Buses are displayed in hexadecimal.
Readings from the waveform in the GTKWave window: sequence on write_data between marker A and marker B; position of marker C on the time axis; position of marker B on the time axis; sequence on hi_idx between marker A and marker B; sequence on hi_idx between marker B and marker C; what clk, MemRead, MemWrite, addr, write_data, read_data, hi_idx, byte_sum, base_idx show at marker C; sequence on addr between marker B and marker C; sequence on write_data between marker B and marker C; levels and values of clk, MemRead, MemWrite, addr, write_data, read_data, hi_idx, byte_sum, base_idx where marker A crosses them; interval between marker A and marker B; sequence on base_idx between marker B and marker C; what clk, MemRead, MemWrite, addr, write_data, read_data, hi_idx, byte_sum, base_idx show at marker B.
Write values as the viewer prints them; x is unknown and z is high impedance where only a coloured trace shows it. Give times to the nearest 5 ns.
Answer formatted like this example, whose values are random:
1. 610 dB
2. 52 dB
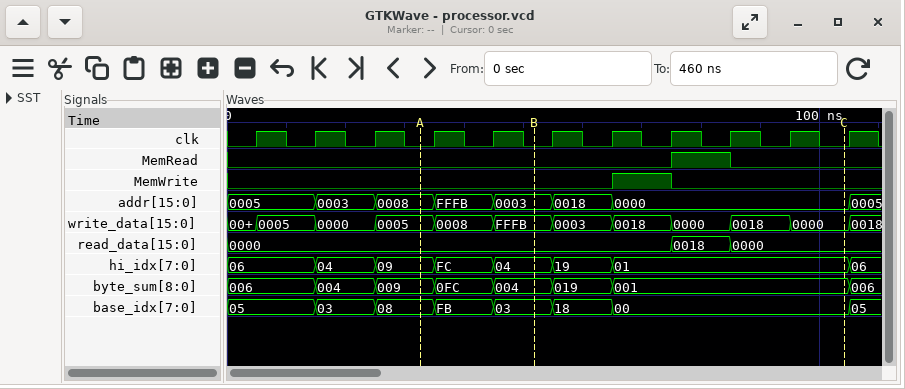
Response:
1. 0005, 0008, FFFB
2. 105 ns
3. 50 ns
4. 09, FC, 04
5. 04, 19, 01
6. clk=0, MemRead=0, MemWrite=0, addr=0000, write_data=0000, read_data=0000, hi_idx=01, byte_sum=001, base_idx=00
7. 0003, 0018, 0000
8. FFFB, 0003, 0018, 0000, 0018, 0000
9. clk=0, MemRead=0, MemWrite=0, addr=0008, write_data=0005, read_data=0000, hi_idx=09, byte_sum=009, base_idx=08
10. 20 ns
11. 03, 18, 00
12. clk=0, MemRead=0, MemWrite=0, addr=0003, write_data=FFFB, read_data=0000, hi_idx=04, byte_sum=004, base_idx=03
